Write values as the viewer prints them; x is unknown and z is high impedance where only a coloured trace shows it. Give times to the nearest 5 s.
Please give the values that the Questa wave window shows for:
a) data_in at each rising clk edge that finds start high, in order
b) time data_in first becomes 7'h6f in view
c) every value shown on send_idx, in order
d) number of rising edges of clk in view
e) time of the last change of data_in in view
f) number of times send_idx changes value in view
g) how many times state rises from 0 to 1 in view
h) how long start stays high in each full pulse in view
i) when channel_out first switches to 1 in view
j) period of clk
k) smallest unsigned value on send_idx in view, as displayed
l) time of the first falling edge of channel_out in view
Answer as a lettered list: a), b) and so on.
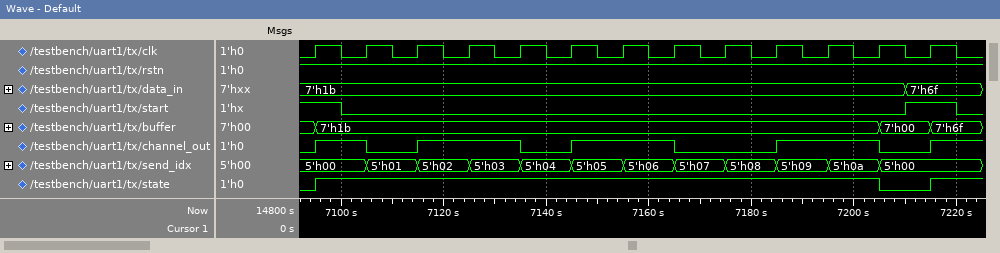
a) 7'h1b, 7'h6f
b) 7210 s
c) 5'h00, 5'h01, 5'h02, 5'h03, 5'h04, 5'h05, 5'h06, 5'h07, 5'h08, 5'h09, 5'h0a, 5'h00
d) 13
e) 7210 s
f) 11
g) 2
h) 10 s
i) 7095 s
j) 10 s
k) 5'h00
l) 7105 s
